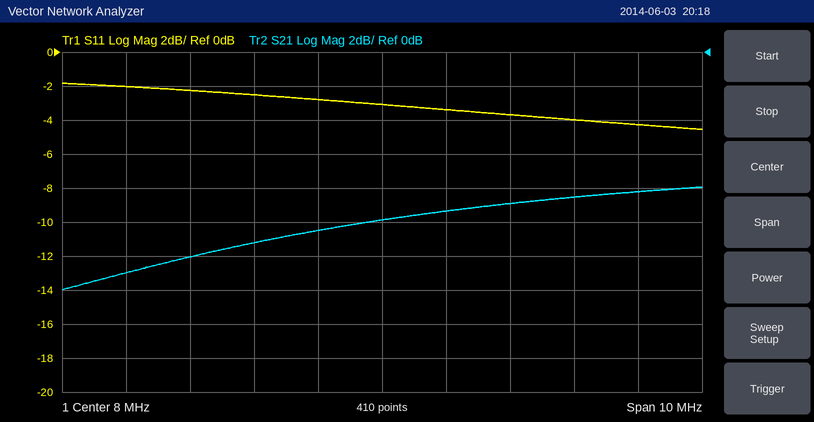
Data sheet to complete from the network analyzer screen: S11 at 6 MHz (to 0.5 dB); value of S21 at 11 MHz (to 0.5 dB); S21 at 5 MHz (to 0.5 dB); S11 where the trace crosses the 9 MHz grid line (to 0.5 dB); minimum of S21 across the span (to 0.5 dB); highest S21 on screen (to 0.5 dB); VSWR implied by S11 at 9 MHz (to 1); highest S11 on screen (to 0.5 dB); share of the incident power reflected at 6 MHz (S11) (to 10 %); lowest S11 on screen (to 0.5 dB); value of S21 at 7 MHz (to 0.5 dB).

-2.5 dB
-8.5 dB
-12.0 dB
-3.5 dB
-14.0 dB
-8.0 dB
5
-2.0 dB
60 %
-4.5 dB
-10.5 dB
